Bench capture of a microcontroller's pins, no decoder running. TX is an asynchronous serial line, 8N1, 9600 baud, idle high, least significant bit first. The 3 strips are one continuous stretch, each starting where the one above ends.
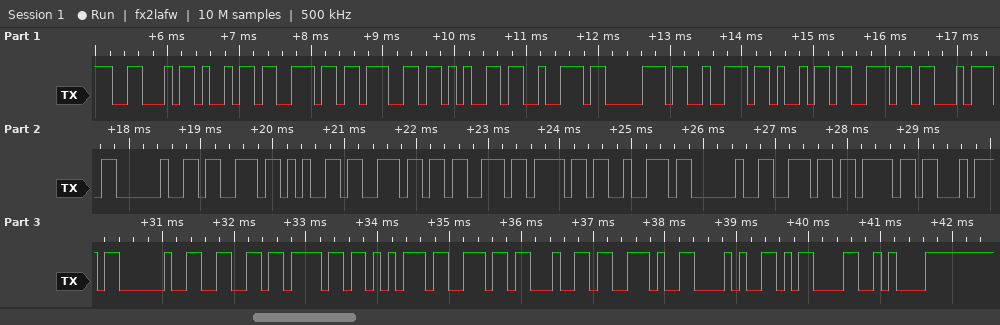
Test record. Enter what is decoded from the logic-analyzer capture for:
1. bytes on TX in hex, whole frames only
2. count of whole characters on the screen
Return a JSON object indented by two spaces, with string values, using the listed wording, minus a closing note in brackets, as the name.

{
  "bytes on TX in hex, whole frames only": "0x46 0x69 0x6E 0x67 0x65 0x72 0x70 0x72 0x69 0x6E 0x74 0x20 0x73 0x65 0x6E 0x73 0x6F 0x72 0x20 0x6E 0x6F 0x74 0x20 0x66 0x6F 0x75 0x6E 0x64 0x2E 0x28 0x0D 0x0A",
  "count of whole characters on the screen": "32"
}
